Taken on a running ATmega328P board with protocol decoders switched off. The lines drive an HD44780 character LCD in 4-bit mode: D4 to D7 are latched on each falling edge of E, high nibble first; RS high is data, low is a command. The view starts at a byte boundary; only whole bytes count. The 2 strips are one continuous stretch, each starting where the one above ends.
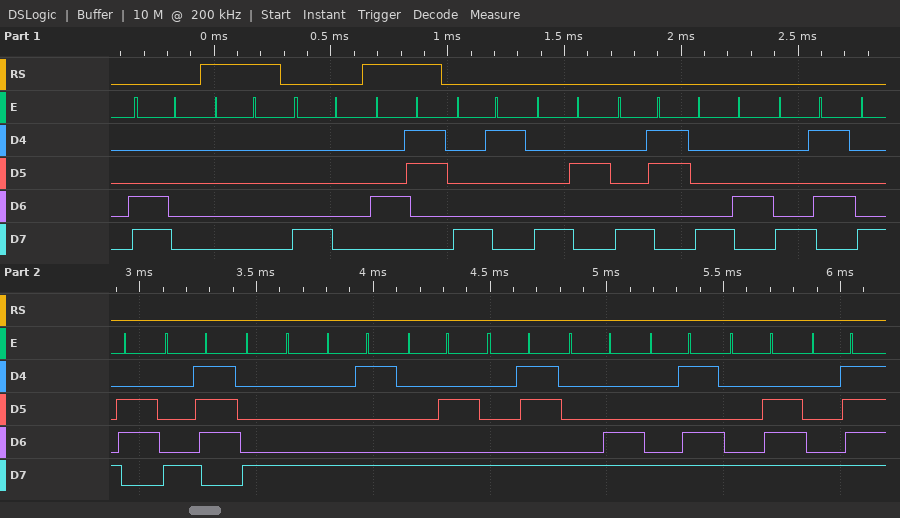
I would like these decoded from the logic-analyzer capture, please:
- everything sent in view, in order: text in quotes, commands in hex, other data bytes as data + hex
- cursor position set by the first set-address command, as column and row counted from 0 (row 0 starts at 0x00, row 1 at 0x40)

0xC0 data 00 0x80 "C" 0x81 0x82 0x83 0x84 0x85 0x86 0x87 0x88 0x89 0x8A 0x8B 0x8C 0x8D 0x8E 0x8F
column 0, row 1
